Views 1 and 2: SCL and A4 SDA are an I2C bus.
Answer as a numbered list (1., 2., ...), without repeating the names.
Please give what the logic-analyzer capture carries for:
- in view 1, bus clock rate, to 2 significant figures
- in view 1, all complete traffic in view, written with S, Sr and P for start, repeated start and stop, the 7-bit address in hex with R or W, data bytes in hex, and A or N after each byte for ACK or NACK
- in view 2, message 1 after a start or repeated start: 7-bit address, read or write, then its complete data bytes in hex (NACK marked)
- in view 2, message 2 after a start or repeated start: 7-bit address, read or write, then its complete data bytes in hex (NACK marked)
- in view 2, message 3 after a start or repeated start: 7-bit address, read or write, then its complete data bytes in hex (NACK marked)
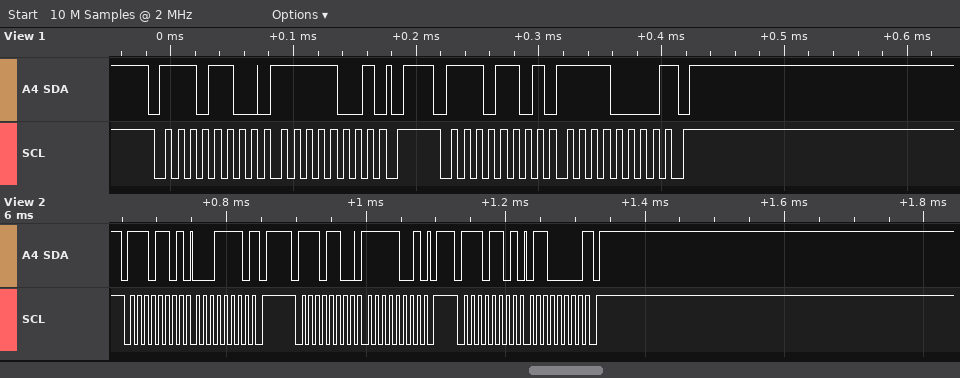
1. 100 kHz
2. S 76W A F9 A P S 76R A F0 N P
3. 0x76 read: 1E NACK
4. 0x76 write: F9
5. 0x76 read: 60 NACK
